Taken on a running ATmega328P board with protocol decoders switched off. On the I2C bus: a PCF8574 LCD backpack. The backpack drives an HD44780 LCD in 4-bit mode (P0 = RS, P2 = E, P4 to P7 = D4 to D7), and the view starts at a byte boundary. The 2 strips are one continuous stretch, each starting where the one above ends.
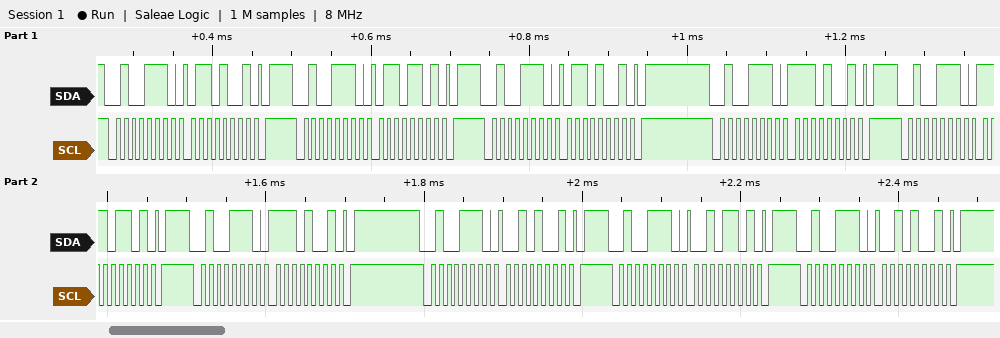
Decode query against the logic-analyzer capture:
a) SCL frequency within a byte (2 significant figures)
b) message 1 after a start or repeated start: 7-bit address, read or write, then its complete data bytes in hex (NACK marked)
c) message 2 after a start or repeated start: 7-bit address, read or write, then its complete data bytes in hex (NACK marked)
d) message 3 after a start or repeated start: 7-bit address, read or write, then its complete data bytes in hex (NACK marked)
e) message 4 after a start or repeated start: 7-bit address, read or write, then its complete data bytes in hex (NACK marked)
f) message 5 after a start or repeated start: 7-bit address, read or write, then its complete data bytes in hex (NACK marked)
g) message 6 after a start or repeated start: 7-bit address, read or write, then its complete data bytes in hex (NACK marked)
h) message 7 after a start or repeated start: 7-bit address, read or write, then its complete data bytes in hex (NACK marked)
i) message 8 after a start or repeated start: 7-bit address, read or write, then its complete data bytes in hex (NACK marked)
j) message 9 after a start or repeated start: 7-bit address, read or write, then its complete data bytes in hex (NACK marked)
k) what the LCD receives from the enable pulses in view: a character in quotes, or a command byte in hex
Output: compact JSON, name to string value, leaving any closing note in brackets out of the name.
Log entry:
{"SCL frequency within a byte": "100 kHz", "message 1 after a start or repeated start: 7-bit address, read or write, then its complete data bytes in hex": "0x27 write: 69", "message 2 after a start or repeated start: 7-bit address, read or write, then its complete data bytes in hex": "0x27 write: 6D", "message 3 after a start or repeated start: 7-bit address, read or write, then its complete data bytes in hex": "0x27 write: 69", "message 4 after a start or repeated start: 7-bit address, read or write, then its complete data bytes in hex": "0x27 write: E9", "message 5 after a start or repeated start: 7-bit address, read or write, then its complete data bytes in hex": "0x27 write: ED", "message 6 after a start or repeated start: 7-bit address, read or write, then its complete data bytes in hex": "0x27 write: E9", "message 7 after a start or repeated start: 7-bit address, read or write, then its complete data bytes in hex": "0x27 write: 29", "message 8 after a start or repeated start: 7-bit address, read or write, then its complete data bytes in hex": "0x27 write: 2D", "message 9 after a start or repeated start: 7-bit address, read or write, then its complete data bytes in hex": "0x27 write: 29", "what the LCD receives from the enable pulses in view: a character in quotes, or a command byte in hex": "'n'"}
